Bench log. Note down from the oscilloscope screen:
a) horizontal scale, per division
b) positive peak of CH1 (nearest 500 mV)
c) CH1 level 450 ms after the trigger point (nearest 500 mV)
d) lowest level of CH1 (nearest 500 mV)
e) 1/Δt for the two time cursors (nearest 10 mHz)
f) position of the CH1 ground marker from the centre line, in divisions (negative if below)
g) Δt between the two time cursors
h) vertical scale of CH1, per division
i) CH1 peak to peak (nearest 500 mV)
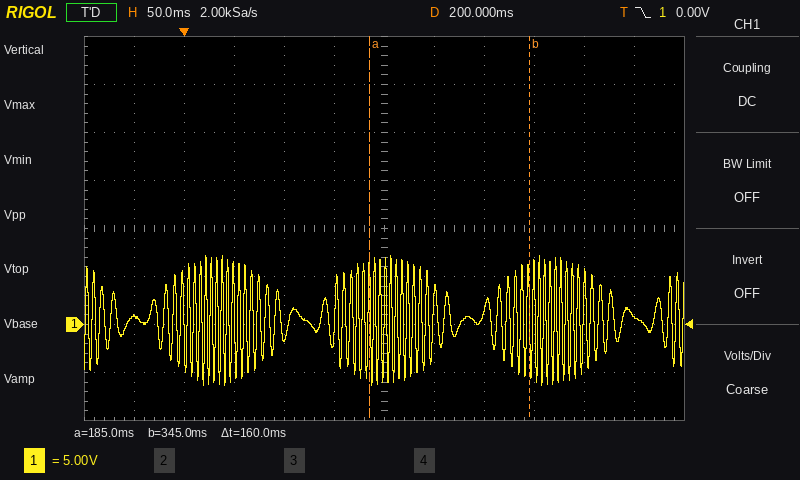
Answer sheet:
50 ms
7.0 V
1.0 V
-6.5 V
6.25 Hz
-2.0 div
160 ms
5 V
13.5 V
